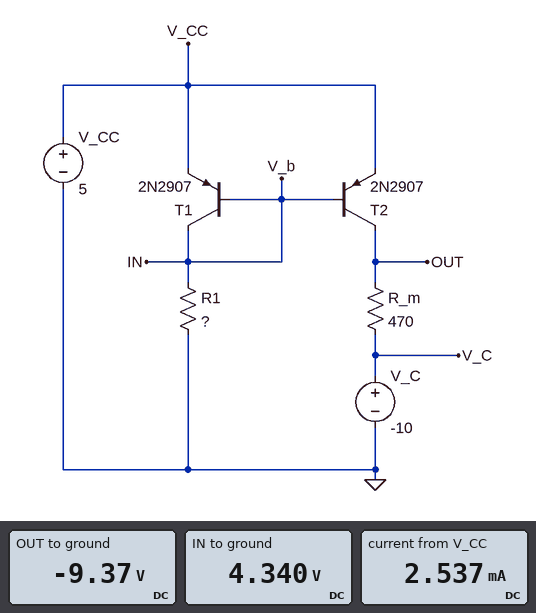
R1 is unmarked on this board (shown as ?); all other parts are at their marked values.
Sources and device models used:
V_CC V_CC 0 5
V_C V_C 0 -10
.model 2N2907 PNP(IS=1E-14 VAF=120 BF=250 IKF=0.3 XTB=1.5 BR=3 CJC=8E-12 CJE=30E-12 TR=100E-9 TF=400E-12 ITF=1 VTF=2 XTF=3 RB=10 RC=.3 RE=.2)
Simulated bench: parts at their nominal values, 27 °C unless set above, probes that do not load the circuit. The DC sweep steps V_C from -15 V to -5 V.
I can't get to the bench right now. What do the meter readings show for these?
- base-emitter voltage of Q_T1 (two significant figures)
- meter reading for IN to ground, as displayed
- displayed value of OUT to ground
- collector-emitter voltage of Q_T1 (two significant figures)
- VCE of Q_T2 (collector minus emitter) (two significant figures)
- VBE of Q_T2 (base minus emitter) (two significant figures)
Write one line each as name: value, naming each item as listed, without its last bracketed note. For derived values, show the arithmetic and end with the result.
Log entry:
base-emitter voltage of Q_T1: 4.34 V - 5 V = -660 mV
meter reading for IN to ground, as displayed: 4.340 V
displayed value of OUT to ground: -9.37 V
collector-emitter voltage of Q_T1: 4.34 V - 5 V = -660 mV
VCE of Q_T2 (collector minus emitter): -9.37 V - 5 V = -14 V
VBE of Q_T2 (base minus emitter): 4.34 V - 5 V = -660 mV
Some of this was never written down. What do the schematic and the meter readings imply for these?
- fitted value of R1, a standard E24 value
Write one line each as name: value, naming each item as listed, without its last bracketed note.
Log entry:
fitted value of R1, a standard E24 value: 3.6 kΩ
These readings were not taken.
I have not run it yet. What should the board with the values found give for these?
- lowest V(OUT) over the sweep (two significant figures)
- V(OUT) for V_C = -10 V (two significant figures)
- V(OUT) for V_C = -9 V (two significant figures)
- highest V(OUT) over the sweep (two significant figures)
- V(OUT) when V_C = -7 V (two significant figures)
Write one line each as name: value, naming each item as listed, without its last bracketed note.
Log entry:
lowest V(OUT) over the sweep: -14 V
V(OUT) for V_C = -10 V: -9.4 V
V(OUT) for V_C = -9 V: -8.4 V
highest V(OUT) over the sweep: -4.4 V
V(OUT) when V_C = -7 V: -6.4 V
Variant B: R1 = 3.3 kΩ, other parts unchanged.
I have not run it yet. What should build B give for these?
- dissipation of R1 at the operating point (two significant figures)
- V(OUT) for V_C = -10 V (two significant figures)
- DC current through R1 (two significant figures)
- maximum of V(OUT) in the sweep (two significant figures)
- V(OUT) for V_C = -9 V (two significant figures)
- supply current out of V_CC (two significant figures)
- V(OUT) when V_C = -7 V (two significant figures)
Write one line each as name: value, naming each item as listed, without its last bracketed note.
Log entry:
dissipation of R1 at the operating point: 5.7 mW
V(OUT) for V_C = -10 V: -9.3 V
DC current through R1: 1.3 mA
maximum of V(OUT) in the sweep: -4.3 V
V(OUT) for V_C = -9 V: -8.3 V
supply current out of V_CC: 2.8 mA
V(OUT) when V_C = -7 V: -6.3 V
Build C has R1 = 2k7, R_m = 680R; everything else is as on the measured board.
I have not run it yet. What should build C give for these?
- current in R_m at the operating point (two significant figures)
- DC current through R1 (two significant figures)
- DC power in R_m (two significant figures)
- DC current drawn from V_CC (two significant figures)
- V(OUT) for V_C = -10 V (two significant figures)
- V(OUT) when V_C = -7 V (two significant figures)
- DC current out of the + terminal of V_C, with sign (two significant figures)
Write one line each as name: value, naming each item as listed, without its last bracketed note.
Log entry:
current in R_m at the operating point: 1.8 mA
DC current through R1: 1.6 mA
DC power in R_m: 2.1 mW
DC current drawn from V_CC: 3.4 mA
V(OUT) for V_C = -10 V: -8.8 V
V(OUT) when V_C = -7 V: -5.8 V
DC current out of the + terminal of V_C, with sign: -1.8 mA
